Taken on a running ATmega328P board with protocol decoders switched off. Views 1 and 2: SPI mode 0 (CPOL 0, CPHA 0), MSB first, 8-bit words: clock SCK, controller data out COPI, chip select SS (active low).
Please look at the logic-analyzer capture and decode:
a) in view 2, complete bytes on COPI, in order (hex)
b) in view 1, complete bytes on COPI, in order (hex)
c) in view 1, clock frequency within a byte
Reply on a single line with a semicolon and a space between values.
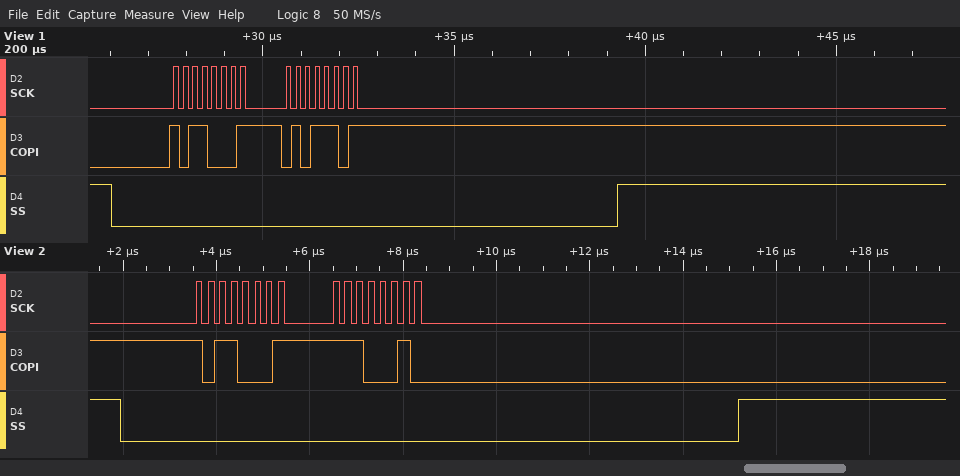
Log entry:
B1 E2; 0xB1 0x5D; 4 MHz
